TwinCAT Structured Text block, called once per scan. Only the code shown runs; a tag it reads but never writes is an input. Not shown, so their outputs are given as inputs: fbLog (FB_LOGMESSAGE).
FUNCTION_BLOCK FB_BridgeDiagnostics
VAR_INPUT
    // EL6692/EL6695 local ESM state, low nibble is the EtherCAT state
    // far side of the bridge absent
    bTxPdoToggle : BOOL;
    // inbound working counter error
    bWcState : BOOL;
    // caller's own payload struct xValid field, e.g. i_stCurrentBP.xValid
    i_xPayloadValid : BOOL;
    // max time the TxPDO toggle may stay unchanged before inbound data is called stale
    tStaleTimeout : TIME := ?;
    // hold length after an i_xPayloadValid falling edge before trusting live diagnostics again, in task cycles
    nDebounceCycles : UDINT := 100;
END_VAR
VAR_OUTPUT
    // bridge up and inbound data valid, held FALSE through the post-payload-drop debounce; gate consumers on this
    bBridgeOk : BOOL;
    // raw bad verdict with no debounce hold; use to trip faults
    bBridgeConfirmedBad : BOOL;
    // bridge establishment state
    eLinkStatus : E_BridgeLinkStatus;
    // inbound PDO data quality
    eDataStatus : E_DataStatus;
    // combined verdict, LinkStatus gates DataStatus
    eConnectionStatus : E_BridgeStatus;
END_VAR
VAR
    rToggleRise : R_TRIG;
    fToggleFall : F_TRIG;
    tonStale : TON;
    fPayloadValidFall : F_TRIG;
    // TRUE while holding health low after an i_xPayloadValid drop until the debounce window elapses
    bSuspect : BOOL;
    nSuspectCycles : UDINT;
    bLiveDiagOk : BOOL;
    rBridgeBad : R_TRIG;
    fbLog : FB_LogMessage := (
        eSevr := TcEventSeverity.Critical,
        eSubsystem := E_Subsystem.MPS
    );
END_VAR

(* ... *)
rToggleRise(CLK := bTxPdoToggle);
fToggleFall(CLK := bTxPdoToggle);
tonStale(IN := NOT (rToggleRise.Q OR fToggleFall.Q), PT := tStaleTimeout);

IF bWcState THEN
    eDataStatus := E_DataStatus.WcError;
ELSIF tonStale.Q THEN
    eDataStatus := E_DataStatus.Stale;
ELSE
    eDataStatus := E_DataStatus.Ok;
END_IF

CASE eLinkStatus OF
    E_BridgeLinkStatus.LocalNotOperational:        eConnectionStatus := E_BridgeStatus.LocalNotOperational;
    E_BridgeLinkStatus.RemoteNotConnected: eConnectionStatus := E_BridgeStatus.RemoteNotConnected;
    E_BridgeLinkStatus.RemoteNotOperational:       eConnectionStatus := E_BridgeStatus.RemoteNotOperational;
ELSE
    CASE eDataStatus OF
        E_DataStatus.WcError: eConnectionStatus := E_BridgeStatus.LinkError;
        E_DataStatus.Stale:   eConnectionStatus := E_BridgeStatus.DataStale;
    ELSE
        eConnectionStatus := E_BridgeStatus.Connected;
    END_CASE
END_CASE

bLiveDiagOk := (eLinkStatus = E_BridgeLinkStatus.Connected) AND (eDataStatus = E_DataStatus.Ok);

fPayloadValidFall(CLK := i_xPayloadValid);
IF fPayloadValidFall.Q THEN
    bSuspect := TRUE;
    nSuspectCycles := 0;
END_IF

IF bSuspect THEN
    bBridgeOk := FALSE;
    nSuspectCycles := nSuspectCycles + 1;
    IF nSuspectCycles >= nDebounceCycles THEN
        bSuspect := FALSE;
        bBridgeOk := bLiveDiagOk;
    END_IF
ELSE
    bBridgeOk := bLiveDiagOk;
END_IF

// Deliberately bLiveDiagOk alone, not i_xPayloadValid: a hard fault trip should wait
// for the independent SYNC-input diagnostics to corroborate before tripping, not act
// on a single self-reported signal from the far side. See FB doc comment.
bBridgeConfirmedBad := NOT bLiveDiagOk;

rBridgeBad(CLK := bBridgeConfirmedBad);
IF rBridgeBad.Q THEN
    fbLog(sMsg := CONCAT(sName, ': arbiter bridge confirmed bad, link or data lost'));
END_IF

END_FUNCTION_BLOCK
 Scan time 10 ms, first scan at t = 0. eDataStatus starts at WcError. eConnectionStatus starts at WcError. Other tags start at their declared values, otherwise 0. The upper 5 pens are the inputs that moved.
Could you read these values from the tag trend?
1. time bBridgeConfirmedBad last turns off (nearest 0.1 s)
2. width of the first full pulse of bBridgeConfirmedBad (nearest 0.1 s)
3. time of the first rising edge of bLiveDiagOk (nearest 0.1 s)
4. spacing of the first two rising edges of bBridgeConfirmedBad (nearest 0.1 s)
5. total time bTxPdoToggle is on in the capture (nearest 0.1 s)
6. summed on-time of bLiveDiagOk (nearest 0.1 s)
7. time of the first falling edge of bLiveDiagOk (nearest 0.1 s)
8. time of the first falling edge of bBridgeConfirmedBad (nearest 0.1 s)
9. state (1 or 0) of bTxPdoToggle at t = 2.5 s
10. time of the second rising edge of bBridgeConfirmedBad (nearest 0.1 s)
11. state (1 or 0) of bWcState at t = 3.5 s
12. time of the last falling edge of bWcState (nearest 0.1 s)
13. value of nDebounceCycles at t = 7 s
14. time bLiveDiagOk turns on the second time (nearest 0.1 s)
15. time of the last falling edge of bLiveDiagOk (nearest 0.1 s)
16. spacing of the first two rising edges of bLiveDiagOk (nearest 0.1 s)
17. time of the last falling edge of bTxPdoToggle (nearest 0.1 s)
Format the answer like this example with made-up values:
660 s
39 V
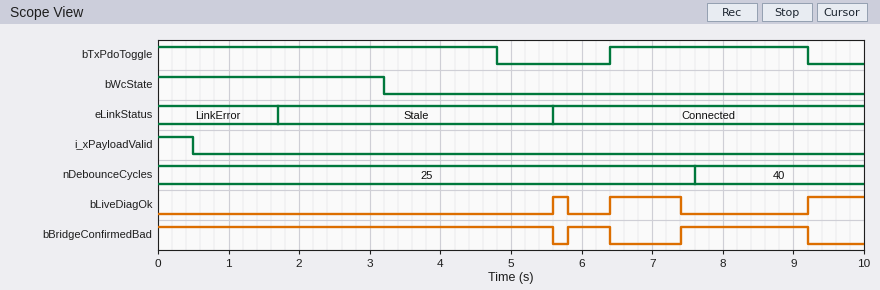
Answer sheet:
9.2 s
0.6 s
5.6 s
1.6 s
7.6 s
2.0 s
5.8 s
5.6 s
1
7.4 s
0
3.2 s
25
6.4 s
7.4 s
0.8 s
9.2 s
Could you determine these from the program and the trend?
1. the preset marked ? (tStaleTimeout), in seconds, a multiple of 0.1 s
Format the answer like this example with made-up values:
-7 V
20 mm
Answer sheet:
1.0 s
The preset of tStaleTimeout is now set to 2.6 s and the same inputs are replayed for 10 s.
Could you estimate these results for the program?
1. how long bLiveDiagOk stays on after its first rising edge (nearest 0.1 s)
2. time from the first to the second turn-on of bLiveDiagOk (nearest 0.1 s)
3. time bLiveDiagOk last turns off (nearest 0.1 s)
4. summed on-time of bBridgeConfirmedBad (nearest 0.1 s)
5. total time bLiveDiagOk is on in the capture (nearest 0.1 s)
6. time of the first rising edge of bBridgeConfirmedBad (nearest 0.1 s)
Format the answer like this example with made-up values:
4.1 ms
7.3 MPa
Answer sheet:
3.4 s
3.6 s
9.0 s
5.8 s
4.2 s
9.0 s
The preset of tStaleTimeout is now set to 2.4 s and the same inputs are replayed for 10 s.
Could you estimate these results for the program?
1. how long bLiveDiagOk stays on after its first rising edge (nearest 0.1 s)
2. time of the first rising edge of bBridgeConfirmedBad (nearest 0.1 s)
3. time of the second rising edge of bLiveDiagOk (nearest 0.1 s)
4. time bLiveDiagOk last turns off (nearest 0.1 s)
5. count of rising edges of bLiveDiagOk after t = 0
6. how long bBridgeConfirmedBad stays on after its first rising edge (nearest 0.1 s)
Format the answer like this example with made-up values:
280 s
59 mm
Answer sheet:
3.2 s
8.8 s
9.2 s
8.8 s
2
0.4 s
